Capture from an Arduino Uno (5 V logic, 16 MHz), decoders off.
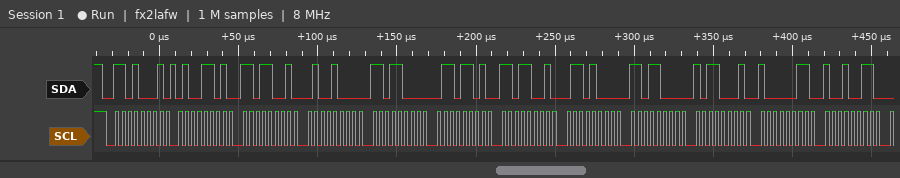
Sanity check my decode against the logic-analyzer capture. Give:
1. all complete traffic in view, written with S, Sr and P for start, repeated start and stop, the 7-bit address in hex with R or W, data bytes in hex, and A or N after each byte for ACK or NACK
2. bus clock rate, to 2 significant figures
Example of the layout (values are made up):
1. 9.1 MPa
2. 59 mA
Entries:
1. S 68R A 4D A D9 A 48 A D8 A 6D A D9 A 68 A D8 A B1 A 83 A 93 A
2. 250 kHz
